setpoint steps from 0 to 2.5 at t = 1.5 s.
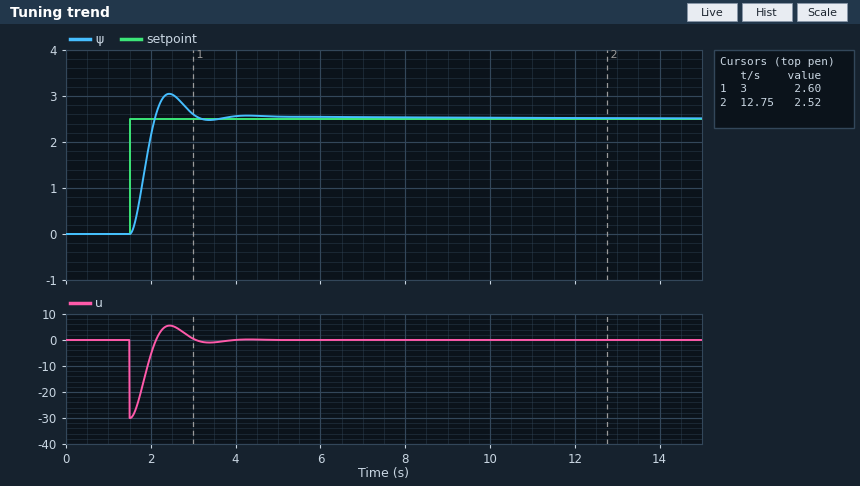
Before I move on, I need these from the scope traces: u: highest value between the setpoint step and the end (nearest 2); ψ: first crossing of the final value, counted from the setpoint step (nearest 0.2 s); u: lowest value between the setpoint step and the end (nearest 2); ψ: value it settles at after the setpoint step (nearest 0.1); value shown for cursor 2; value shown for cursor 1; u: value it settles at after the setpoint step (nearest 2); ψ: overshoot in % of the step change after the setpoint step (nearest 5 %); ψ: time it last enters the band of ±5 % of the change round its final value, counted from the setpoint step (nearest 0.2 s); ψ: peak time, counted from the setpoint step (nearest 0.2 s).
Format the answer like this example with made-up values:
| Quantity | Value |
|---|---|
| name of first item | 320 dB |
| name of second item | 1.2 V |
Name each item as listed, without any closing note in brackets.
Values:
| Quantity | Value |
|---|---|
| u: highest value between the setpoint step and the end | 6 |
| ψ: first crossing of the final value, counted from the setpoint step | 0.6 s |
| u: lowest value between the setpoint step and the end | -30 |
| ψ: value it settles at after the setpoint step | 2.5 |
| value shown for cursor 2 | 2.52 |
| value shown for cursor 1 | 2.60 |
| u: value it settles at after the setpoint step | 0 |
| ψ: overshoot in % of the step change after the setpoint step | 20 % |
| ψ: time it last enters the band of ±5 % of the change round its final value, counted from the setpoint step | 1.4 s |
| ψ: peak time, counted from the setpoint step | 1.0 s |
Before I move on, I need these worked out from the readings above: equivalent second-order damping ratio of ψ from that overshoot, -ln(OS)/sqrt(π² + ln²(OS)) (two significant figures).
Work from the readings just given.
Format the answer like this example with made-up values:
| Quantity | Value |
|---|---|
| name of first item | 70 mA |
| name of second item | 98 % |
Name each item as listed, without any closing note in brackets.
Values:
| Quantity | Value |
|---|---|
| equivalent second-order damping ratio of ψ from that overshoot, -ln(OS)/sqrt(π² + ln²(OS)) | 0.46 |
